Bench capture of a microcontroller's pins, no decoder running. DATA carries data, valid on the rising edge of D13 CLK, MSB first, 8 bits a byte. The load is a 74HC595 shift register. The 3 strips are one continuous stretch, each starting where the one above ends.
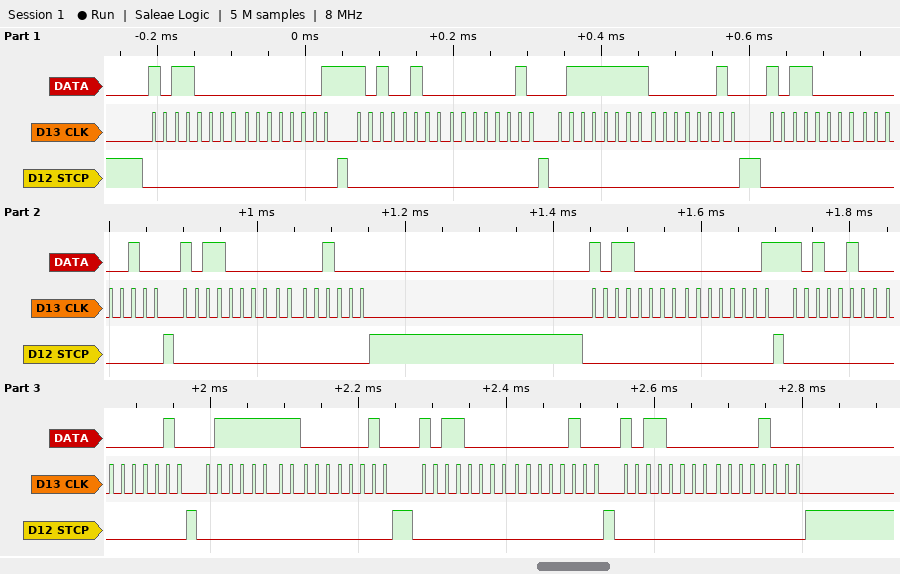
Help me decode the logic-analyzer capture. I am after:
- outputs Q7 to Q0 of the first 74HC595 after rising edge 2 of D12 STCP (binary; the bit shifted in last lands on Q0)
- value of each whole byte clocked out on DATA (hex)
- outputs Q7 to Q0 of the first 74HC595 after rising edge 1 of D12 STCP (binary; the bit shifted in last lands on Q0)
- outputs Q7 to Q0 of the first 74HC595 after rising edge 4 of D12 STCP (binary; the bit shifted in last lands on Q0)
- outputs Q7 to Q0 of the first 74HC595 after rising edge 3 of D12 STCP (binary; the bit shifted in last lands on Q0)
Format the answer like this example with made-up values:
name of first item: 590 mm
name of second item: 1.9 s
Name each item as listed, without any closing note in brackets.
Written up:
outputs Q7 to Q0 of the first 74HC595 after rising edge 2 of D12 STCP: 00000010
value of each whole byte clocked out on DATA: B0 01 A4 02 7F 02 B0 04 B0 08 B0 01 A4 02 7F 02 B0 04 B0 08
outputs Q7 to Q0 of the first 74HC595 after rising edge 1 of D12 STCP: 00000001
outputs Q7 to Q0 of the first 74HC595 after rising edge 4 of D12 STCP: 00000100
outputs Q7 to Q0 of the first 74HC595 after rising edge 3 of D12 STCP: 00000010
